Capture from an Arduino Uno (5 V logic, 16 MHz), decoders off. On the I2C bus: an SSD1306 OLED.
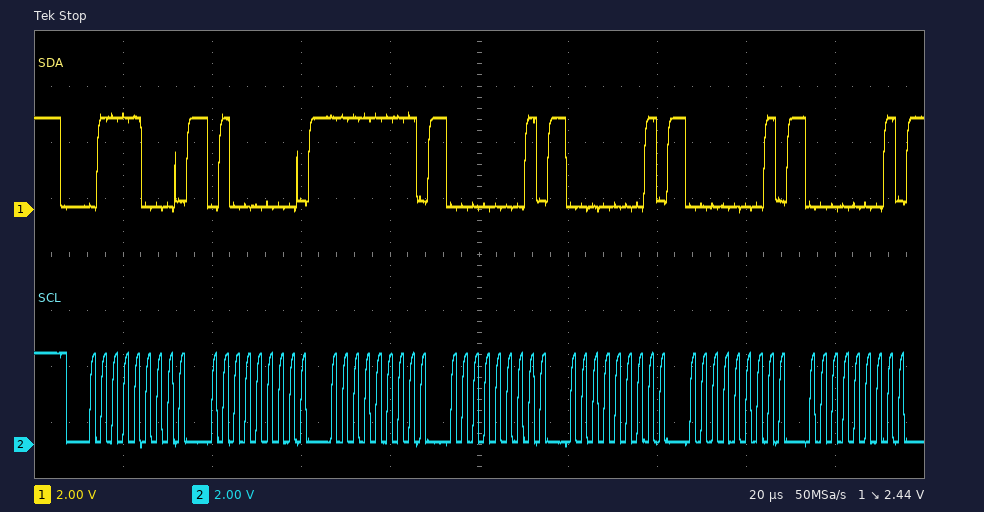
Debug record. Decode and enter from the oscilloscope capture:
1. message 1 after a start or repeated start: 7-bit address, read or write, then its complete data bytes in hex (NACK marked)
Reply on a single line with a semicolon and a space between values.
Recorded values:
0x3C write: 40 FF 01 01 01 01
